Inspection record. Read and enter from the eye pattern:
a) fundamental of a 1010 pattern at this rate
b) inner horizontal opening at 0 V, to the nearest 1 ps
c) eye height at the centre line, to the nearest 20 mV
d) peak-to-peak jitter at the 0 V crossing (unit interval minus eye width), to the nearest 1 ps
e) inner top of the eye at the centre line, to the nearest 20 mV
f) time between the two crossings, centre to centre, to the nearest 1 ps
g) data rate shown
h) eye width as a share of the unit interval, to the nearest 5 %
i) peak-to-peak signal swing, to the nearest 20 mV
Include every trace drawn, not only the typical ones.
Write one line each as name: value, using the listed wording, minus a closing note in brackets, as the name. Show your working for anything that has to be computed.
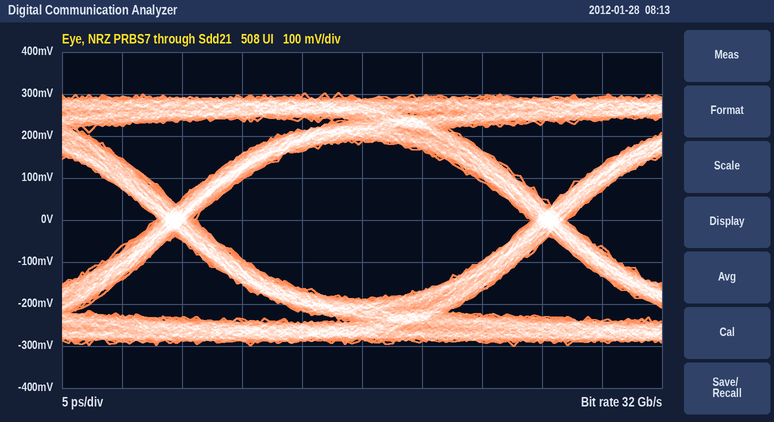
fundamental of a 1010 pattern at this rate: 16 GHz
inner horizontal opening at 0 V, to the nearest 1 ps: 28 ps
eye height at the centre line, to the nearest 20 mV: 380 mV
peak-to-peak jitter at the 0 V crossing (unit interval minus eye width), to the nearest 1 ps: 3 ps
inner top of the eye at the centre line, to the nearest 20 mV: 180 mV
time between the two crossings, centre to centre, to the nearest 1 ps: 31 ps
data rate shown: 32 Gb/s
eye width as a share of the unit interval, to the nearest 5 %: 28 ps / 31 ps ≈ 90 %
peak-to-peak signal swing, to the nearest 20 mV: 600 mV
